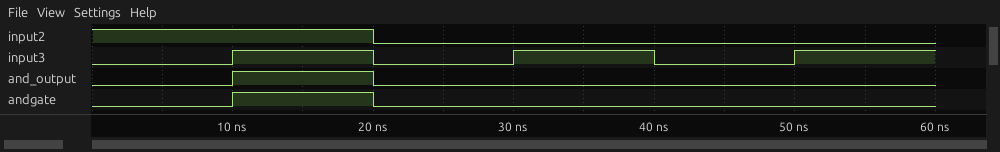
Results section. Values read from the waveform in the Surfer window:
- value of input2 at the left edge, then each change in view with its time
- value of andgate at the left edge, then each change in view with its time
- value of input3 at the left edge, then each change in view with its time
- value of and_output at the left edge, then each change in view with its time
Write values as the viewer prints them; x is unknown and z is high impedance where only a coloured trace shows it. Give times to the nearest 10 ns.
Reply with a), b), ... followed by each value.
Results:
a) 1, 0 at 20 ns
b) 0, 1 at 10 ns, 0 at 20 ns
c) 0, 1 at 10 ns, 0 at 20 ns, 1 at 30 ns, 0 at 40 ns, 1 at 50 ns
d) 0, 1 at 10 ns, 0 at 20 ns
